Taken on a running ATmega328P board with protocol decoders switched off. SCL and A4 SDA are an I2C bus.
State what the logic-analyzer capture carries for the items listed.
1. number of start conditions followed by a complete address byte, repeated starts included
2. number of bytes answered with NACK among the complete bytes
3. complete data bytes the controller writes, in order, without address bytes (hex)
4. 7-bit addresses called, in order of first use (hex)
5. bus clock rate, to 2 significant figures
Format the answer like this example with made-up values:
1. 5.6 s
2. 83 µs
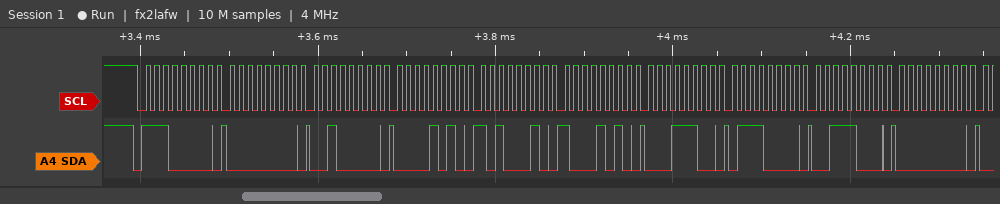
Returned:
1. 1
2. 0
3. 00 20 0A A2 8A 1C 70 38 00
4. 0x70
5. 100 kHz
